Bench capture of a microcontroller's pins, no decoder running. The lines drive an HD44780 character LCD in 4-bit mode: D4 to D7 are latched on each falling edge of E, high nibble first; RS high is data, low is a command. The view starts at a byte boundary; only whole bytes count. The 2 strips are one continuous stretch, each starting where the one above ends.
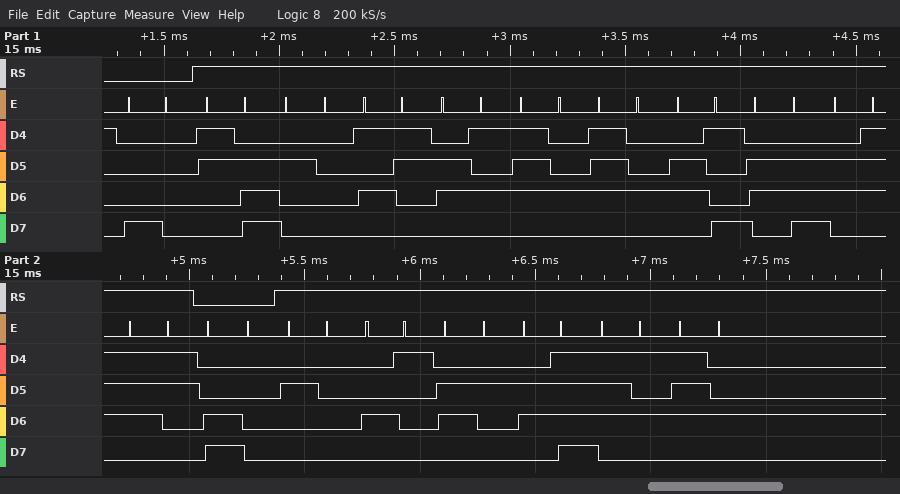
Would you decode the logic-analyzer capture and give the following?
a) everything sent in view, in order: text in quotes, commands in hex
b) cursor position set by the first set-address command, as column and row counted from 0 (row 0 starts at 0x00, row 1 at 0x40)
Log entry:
0x80 "> Settings" 0xC0 " About"
column 0, row 0
